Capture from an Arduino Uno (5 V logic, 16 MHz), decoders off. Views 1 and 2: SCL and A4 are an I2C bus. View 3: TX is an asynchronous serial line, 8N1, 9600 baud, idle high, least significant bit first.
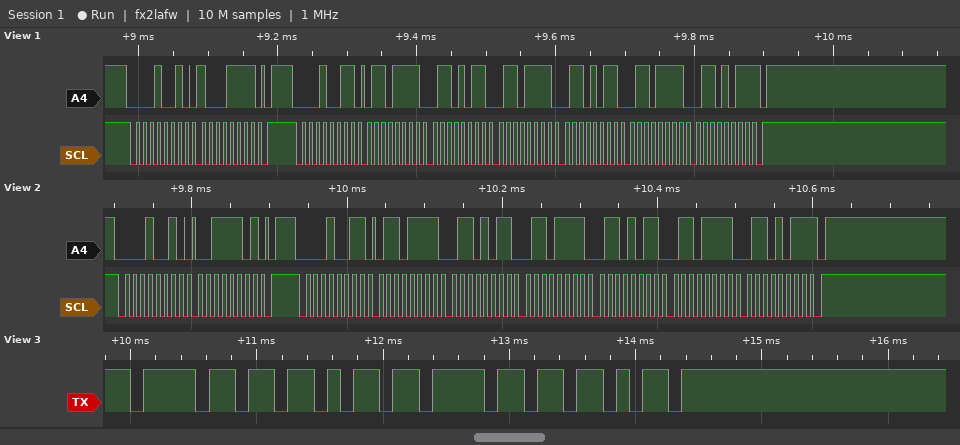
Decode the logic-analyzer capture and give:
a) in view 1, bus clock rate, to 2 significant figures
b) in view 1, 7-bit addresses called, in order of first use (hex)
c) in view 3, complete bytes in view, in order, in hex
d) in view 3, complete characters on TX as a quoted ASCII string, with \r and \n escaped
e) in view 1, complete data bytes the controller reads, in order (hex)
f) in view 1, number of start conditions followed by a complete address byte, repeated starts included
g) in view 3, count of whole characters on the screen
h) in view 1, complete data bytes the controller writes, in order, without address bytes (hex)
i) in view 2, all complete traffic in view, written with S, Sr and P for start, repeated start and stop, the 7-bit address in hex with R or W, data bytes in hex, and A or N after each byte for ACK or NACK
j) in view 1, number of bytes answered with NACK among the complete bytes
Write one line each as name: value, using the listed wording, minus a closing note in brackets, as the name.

in view 1, bus clock rate, to 2 significant figures: 100 kHz
in view 1, 7-bit addresses called, in order of first use: 0x09
in view 3, complete bytes in view, in order, in hex: 6F 6B 6F 6B
in view 3, complete characters on TX as a quoted ASCII string, with \r and \n escaped: "okok"
in view 1, complete data bytes the controller reads, in order: 6F 6B 6F 6B 6F 6B
in view 1, number of start conditions followed by a complete address byte, repeated starts included: 2
in view 3, count of whole characters on the screen: 4
in view 1, complete data bytes the controller writes, in order, without address bytes: 8F
in view 2, all complete traffic in view, written with S, Sr and P for start, repeated start and stop, the 7-bit address in hex with R or W, data bytes in hex, and A or N after each byte for ACK or NACK: S 09W A 3D A P S 09R A 6F A 6B A 6F A 6B A 6F A 6B N P
in view 1, number of bytes answered with NACK among the complete bytes: 1
